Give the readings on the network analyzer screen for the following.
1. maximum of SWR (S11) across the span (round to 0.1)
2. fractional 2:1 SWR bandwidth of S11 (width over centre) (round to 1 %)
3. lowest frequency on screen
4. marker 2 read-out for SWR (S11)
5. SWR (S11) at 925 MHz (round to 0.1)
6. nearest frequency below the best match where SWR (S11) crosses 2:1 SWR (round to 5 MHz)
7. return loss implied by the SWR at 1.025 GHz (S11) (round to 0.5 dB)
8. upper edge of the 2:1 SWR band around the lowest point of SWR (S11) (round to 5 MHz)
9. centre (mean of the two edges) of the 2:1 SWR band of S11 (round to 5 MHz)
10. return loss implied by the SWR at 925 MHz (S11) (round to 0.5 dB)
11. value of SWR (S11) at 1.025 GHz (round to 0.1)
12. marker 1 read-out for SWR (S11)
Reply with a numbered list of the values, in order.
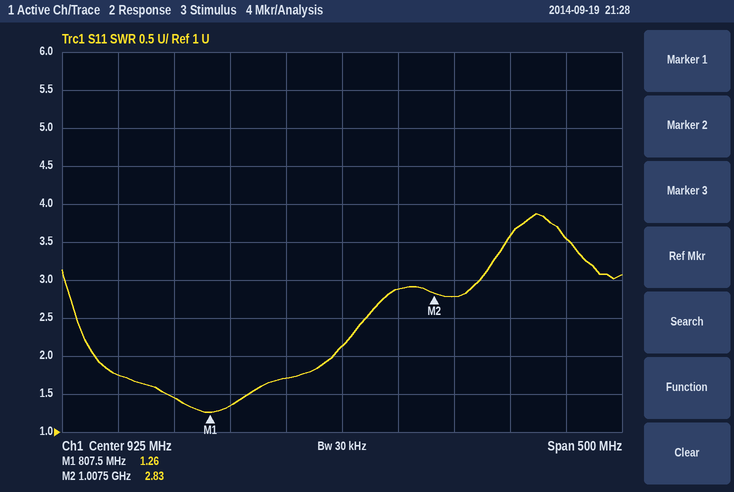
1. 3.9
2. 26 %
3. 675 MHz
4. 2.83
5. 2.1
6. 705 MHz
7. 6.5 dB
8. 915 MHz
9. 810 MHz
10. 9.0 dB
11. 2.8
12. 1.26
